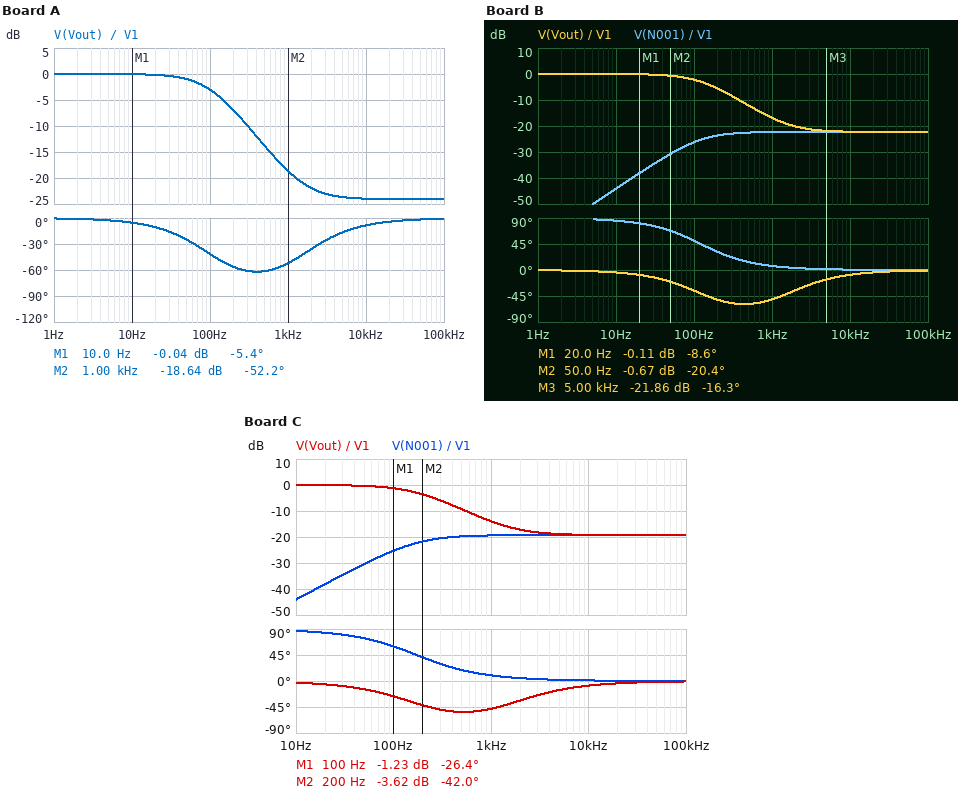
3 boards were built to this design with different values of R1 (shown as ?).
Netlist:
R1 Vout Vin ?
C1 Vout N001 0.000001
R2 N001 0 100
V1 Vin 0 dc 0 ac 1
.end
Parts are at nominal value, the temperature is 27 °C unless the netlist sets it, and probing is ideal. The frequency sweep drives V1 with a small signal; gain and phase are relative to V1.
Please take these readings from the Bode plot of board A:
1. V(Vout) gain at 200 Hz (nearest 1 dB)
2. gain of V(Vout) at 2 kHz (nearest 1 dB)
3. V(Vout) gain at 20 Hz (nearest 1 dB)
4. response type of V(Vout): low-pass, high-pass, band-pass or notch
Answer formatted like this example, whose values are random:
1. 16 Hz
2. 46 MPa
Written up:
1. -7 dB
2. -22 dB
3. 0 dB
4. low-pass
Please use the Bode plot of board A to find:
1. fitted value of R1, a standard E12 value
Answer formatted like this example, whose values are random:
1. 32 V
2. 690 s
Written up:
1. 1.5 kΩ
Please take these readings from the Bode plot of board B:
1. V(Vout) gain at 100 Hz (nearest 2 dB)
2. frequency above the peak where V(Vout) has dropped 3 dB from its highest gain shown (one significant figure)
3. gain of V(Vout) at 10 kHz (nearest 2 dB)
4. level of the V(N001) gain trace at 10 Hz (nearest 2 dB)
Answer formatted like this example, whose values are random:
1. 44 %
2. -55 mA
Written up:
1. -2 dB
2. 100 Hz
3. -22 dB
4. -44 dB
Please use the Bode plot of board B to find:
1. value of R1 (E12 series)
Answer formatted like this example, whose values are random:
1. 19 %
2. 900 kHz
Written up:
1. 1.2 kΩ
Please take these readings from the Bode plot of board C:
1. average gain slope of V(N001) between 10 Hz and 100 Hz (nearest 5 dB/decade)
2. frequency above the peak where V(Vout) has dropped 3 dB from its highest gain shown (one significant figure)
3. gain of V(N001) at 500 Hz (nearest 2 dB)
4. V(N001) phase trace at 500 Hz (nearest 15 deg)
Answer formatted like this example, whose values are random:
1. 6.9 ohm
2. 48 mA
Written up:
1. 20 dB/decade
2. 200 Hz
3. -20 dB
4. 15 deg
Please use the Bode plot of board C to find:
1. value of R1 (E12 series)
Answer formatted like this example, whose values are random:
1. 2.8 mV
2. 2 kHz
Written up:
1. 820 Ω
